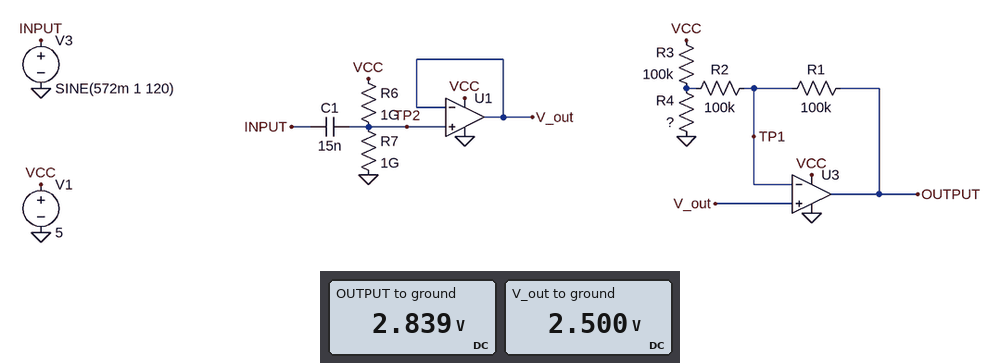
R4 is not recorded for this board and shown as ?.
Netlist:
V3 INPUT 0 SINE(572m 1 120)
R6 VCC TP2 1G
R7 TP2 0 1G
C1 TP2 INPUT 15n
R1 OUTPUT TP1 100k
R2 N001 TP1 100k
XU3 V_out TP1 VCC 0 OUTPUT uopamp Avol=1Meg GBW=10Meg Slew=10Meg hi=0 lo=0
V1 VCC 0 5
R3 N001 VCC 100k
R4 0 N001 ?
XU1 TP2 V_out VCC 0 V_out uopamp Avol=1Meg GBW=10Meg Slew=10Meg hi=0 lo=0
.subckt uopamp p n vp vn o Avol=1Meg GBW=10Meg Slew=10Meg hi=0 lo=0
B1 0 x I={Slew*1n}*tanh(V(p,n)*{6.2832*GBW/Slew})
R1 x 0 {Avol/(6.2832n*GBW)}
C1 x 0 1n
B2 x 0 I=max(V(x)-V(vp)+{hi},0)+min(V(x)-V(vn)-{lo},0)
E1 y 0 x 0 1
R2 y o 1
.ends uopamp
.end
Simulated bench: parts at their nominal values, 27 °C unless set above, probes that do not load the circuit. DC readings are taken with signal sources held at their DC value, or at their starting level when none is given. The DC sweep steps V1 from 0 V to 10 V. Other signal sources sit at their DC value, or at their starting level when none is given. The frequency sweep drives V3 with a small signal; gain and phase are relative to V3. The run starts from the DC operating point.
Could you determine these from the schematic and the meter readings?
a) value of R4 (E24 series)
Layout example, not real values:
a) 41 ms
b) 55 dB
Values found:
a) 68 kΩ
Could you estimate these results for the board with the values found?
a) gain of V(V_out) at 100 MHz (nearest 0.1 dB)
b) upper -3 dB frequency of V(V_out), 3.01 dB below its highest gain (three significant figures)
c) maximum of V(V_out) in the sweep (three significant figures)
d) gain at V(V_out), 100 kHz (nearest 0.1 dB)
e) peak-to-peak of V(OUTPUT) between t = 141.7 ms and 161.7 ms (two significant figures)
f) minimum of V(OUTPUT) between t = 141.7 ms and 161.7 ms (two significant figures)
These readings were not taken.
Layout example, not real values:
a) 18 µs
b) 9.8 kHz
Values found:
a) -20.0 dB
b) 10.0 MHz
c) 5.00 V
d) 0 dB
e) 3.4 V
f) 1.1 V
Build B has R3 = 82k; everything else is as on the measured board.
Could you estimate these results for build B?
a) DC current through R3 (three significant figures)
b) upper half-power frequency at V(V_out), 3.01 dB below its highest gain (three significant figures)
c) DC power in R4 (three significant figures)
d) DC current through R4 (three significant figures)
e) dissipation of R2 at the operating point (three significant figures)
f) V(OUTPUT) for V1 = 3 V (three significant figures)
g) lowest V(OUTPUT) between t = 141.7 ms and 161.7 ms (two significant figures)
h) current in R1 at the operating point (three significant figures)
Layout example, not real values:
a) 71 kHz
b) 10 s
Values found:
a) 32.6 µA
b) 10.0 MHz
c) 79.8 µW
d) 34.3 µA
e) 289 nW
f) 1.60 V
g) 940 mV
h) 1.70 µA
